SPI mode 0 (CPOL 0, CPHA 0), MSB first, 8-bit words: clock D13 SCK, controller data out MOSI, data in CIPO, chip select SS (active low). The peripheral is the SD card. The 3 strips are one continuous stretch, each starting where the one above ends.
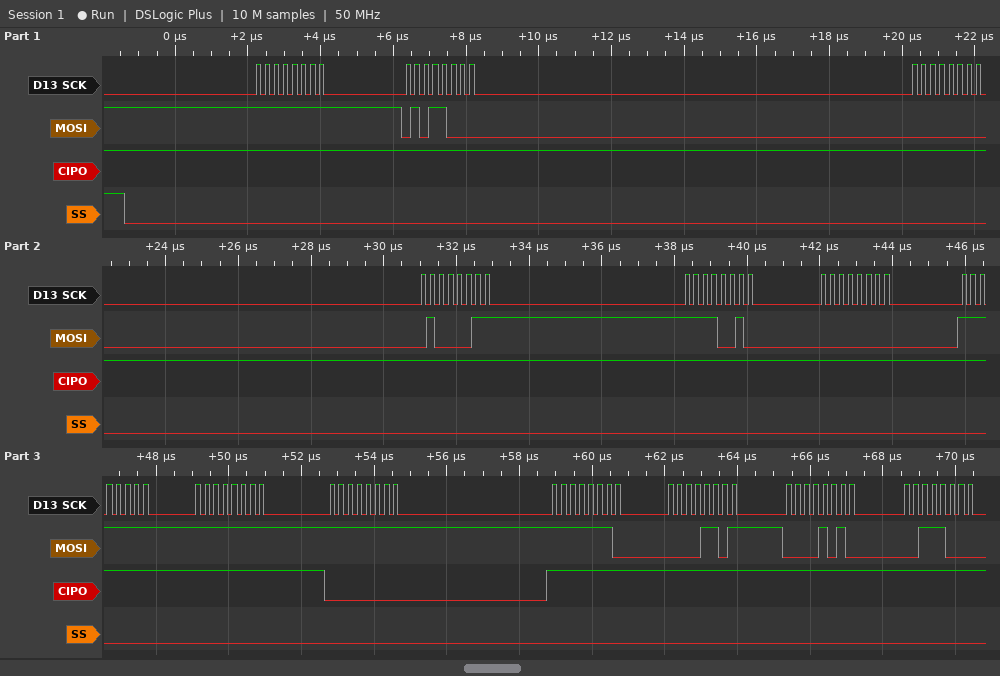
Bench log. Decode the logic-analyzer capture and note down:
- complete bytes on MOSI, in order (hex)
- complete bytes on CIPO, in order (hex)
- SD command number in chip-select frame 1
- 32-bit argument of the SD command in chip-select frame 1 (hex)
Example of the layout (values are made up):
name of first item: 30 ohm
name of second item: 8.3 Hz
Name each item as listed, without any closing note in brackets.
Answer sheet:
complete bytes on MOSI, in order: FF 58 00 43 F2 00 FF FF FF FE 0D 0A 38
complete bytes on CIPO, in order: FF FF FF FF FF FF FF FF 00 FF FF FF FF
SD command number in chip-select frame 1: CMD24
32-bit argument of the SD command in chip-select frame 1: 0x0043F200
